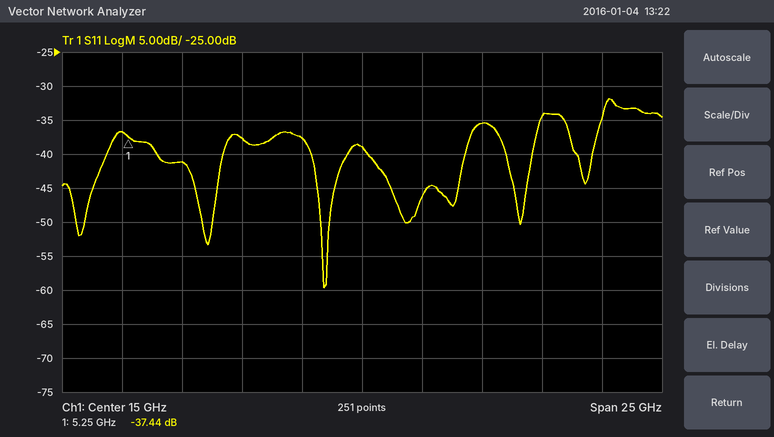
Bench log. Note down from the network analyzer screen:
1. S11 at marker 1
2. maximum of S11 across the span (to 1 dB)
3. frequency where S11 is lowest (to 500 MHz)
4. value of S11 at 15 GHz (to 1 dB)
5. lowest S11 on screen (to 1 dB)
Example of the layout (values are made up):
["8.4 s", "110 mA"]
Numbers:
["-37.44 dB", "-32 dB", "13.5 GHz", "-39 dB", "-60 dB"]
